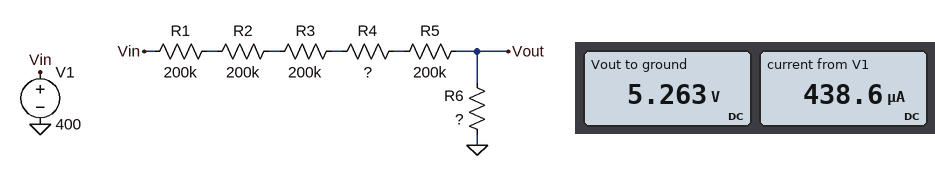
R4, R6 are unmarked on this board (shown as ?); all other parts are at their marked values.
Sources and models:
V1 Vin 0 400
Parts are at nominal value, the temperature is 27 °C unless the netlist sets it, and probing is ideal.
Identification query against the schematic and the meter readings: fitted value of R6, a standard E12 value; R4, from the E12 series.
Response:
12 kΩ
100 kΩ
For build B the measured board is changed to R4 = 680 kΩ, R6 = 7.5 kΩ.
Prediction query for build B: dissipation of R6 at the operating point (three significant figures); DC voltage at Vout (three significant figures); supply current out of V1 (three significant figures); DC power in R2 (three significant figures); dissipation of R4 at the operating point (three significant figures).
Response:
542 µW
2.02 V
269 µA
14.5 mW
49.2 mW
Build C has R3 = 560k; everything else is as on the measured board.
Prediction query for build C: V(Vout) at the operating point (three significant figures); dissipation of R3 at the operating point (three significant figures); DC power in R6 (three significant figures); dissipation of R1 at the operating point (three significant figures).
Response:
3.77 V
55.4 mW
1.19 mW
19.8 mW
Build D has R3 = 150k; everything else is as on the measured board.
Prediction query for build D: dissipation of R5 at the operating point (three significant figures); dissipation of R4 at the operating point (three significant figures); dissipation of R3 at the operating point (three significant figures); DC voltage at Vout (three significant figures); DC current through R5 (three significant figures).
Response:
43.1 mW
21.5 mW
32.3 mW
5.57 V
464 µA
